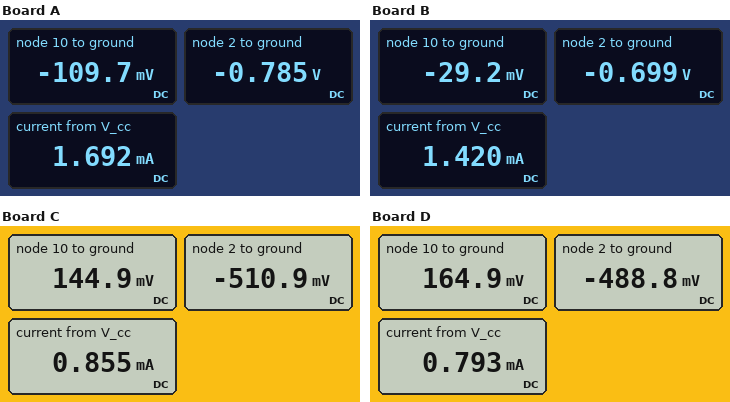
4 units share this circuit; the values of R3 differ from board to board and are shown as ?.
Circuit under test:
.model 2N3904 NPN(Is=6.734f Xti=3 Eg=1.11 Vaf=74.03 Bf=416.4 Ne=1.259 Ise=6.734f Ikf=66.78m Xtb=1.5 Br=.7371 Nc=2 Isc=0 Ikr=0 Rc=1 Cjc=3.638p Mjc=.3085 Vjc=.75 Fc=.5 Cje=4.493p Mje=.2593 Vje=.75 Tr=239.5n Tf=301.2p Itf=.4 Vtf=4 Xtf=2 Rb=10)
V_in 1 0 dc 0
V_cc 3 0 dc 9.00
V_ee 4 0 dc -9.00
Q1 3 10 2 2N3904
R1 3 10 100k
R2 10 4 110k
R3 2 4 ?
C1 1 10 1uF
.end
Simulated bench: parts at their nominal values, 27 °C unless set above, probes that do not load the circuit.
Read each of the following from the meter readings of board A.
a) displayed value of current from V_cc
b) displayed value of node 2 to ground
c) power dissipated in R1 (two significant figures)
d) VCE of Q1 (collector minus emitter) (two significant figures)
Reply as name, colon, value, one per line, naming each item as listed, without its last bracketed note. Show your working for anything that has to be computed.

displayed value of current from V_cc: 1.692 mA
displayed value of node 2 to ground: -0.785 V
power dissipated in R1: (9 V - (-109.7 mV))^2 / 100 kΩ = 830 µW
VCE of Q1 (collector minus emitter): 9 V - (-785 mV) = 9.8 V
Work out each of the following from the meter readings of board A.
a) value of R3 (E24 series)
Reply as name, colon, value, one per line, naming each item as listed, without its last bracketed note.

value of R3: 5.1 kΩ
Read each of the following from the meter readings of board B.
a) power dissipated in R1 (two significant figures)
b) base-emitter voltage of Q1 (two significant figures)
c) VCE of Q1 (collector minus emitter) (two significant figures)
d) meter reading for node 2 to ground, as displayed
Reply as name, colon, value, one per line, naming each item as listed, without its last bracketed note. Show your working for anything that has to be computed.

power dissipated in R1: (9 V - (-29.2 mV))^2 / 100 kΩ = 820 µW
base-emitter voltage of Q1: -29.2 mV - (-699 mV) = 670 mV
VCE of Q1 (collector minus emitter): 9 V - (-699 mV) = 9.7 V
meter reading for node 2 to ground, as displayed: -0.699 V
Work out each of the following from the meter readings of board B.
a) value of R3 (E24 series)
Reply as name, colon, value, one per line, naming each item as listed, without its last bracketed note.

value of R3: 6.2 kΩ
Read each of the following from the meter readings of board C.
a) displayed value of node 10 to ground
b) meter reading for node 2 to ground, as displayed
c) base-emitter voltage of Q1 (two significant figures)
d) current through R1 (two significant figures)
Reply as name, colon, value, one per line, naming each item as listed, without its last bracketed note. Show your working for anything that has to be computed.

displayed value of node 10 to ground: 144.9 mV
meter reading for node 2 to ground, as displayed: -510.9 mV
base-emitter voltage of Q1: 144.9 mV - (-510.9 mV) = 660 mV
current through R1: (9 V - 144.9 mV) / 100 kΩ = 89 µA
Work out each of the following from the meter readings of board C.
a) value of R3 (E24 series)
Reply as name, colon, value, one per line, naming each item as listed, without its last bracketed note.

value of R3: 11 kΩ
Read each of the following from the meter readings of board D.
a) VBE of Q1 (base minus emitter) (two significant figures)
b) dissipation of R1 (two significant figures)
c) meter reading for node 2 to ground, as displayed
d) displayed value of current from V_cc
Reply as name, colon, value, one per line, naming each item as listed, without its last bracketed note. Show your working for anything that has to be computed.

VBE of Q1 (base minus emitter): 164.9 mV - (-488.8 mV) = 650 mV
dissipation of R1: (9 V - 164.9 mV)^2 / 100 kΩ = 780 µW
meter reading for node 2 to ground, as displayed: -488.8 mV
displayed value of current from V_cc: 0.793 mA
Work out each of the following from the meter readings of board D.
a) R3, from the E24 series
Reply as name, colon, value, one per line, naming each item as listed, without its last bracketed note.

R3, from the E24 series: 12 kΩ
